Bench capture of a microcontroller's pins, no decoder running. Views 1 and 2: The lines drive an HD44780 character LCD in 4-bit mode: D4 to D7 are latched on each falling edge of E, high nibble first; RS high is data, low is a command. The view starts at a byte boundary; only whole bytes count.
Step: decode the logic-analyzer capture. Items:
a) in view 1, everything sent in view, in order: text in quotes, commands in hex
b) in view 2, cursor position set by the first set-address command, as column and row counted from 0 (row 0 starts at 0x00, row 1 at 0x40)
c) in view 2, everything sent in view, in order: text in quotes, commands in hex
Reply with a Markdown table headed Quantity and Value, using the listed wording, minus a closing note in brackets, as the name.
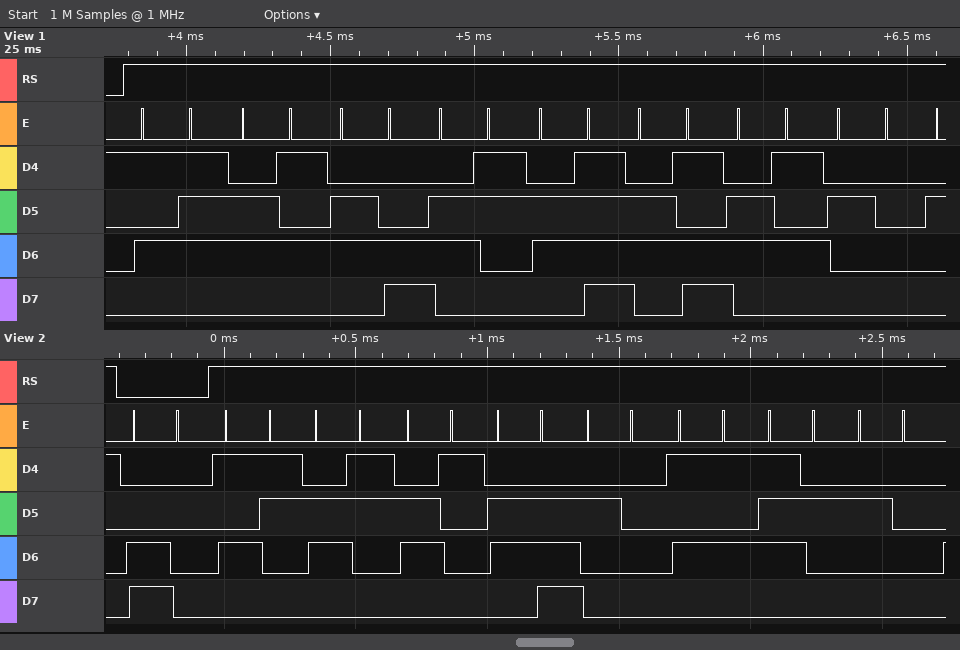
| Quantity | Value |
|---|---|
| in view 1, everything sent in view, in order: text in quotes, commands in hex | "Welcome " |
| in view 2, cursor position set by the first set-address command, as column and row counted from 0 | column 0, row 1 |
| in view 2, everything sent in view, in order: text in quotes, commands in hex | 0xC0 "Scan Ur " |
